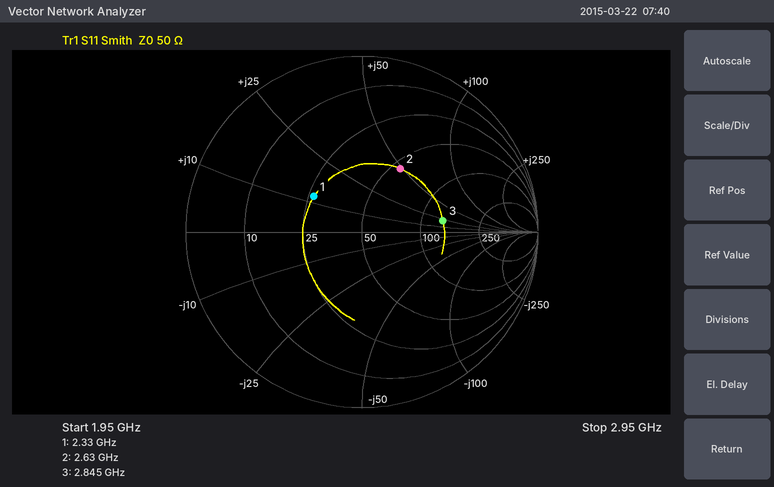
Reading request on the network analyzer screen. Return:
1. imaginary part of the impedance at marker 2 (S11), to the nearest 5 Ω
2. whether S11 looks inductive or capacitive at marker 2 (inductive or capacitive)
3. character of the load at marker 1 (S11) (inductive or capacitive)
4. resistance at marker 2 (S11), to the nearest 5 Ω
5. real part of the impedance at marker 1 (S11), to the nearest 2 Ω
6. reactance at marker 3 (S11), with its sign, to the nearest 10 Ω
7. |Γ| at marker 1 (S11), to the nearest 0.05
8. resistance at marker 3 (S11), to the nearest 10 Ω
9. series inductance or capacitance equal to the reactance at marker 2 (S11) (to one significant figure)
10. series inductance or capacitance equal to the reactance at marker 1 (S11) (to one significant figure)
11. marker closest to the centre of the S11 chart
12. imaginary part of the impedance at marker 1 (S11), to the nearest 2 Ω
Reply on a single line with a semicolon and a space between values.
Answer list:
+50 Ω; inductive; inductive; 55 Ω; 26 Ω; +20 Ω; 0.35; 130 Ω; 3 nH; 800 pH; marker 1; +12 Ω
